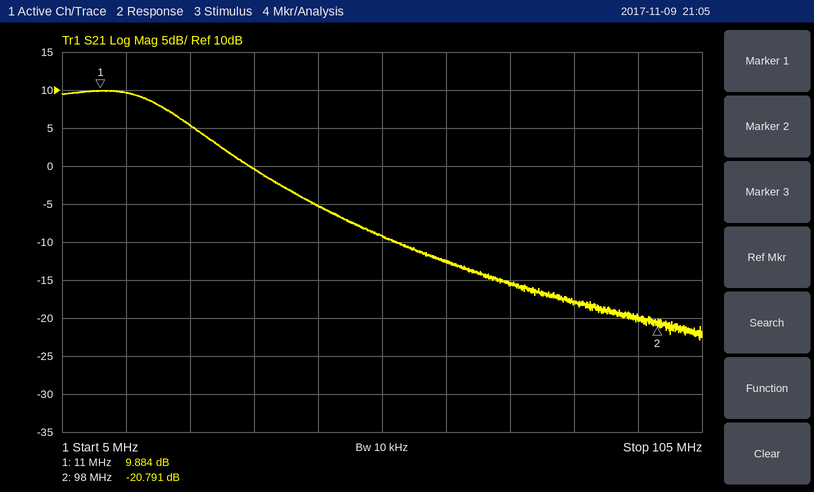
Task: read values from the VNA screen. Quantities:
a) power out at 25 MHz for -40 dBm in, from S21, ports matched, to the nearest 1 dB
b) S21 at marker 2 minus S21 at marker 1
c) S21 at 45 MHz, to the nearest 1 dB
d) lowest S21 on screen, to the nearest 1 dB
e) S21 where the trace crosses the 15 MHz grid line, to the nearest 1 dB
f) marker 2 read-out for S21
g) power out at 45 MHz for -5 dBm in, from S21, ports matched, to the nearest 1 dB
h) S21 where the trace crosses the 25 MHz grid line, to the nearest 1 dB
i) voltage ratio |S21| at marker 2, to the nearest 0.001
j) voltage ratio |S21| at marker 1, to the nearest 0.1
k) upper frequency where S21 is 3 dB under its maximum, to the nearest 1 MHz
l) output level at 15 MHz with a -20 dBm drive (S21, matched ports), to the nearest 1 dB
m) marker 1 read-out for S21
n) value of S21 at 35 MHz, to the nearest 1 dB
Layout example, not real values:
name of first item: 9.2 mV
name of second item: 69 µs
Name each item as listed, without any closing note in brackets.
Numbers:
power out at 25 MHz for -40 dBm in, from S21, ports matched, to the nearest 1 dB: -35 dBm
S21 at marker 2 minus S21 at marker 1: -30.675 dB
S21 at 45 MHz, to the nearest 1 dB: -5 dB
lowest S21 on screen, to the nearest 1 dB: -23 dB
S21 where the trace crosses the 15 MHz grid line, to the nearest 1 dB: 10 dB
marker 2 read-out for S21: -20.791 dB
power out at 45 MHz for -5 dBm in, from S21, ports matched, to the nearest 1 dB: -10 dBm
S21 where the trace crosses the 25 MHz grid line, to the nearest 1 dB: 5 dB
voltage ratio |S21| at marker 2, to the nearest 0.001: 0.091
voltage ratio |S21| at marker 1, to the nearest 0.1: 3.1
upper frequency where S21 is 3 dB under its maximum, to the nearest 1 MHz: 22 MHz
output level at 15 MHz with a -20 dBm drive (S21, matched ports), to the nearest 1 dB: -10 dBm
marker 1 read-out for S21: 9.884 dB
value of S21 at 35 MHz, to the nearest 1 dB: 0 dB
